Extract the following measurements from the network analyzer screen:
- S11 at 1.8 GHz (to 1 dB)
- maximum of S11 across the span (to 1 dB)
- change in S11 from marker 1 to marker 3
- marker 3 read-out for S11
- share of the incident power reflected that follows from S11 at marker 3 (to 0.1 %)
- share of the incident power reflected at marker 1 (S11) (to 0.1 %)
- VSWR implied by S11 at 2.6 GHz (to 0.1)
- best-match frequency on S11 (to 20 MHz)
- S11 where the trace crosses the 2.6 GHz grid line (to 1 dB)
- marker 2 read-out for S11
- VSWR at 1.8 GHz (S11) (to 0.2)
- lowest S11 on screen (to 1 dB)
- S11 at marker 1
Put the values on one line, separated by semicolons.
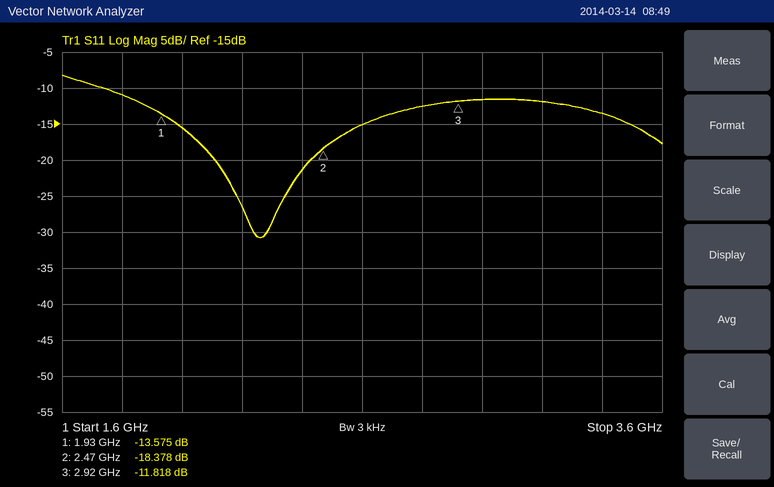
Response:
-11 dB; -8 dB; 1.757 dB; -11.818 dB; 6.6 %; 4.4 %; 1.4; 2.26 GHz; -15 dB; -18.378 dB; 1.8; -31 dB; -13.575 dB
